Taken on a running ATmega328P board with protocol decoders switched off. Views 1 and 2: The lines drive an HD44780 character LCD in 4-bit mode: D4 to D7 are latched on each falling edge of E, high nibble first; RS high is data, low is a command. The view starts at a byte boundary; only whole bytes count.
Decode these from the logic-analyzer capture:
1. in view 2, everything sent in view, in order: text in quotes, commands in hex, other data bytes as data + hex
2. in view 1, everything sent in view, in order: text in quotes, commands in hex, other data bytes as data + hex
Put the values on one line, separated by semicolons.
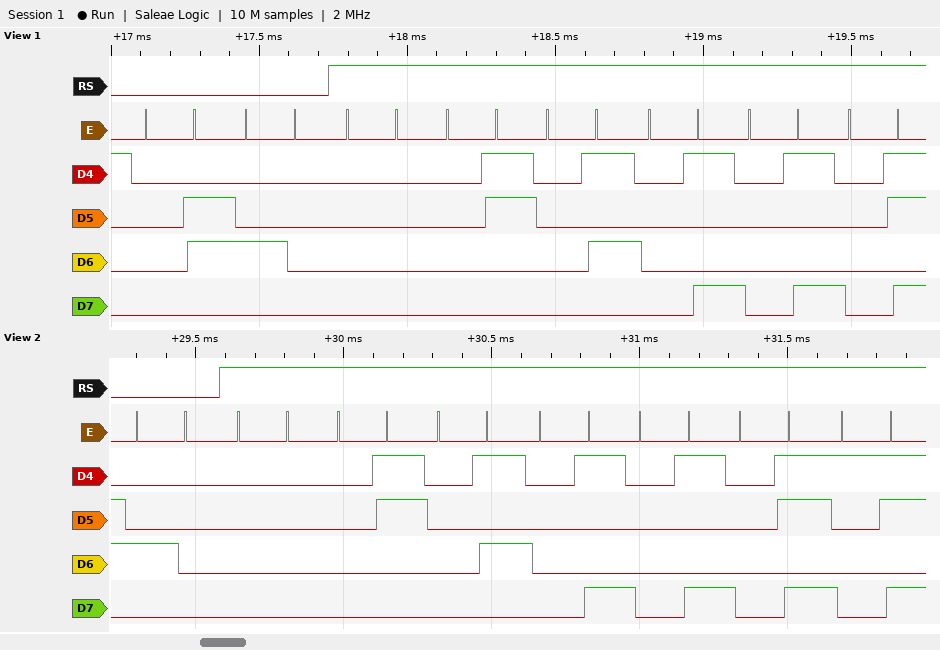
0x40 data 00 03 05 09 09 0B 1B; 0x06 0x40 data 00 03 05 09 09 0B
